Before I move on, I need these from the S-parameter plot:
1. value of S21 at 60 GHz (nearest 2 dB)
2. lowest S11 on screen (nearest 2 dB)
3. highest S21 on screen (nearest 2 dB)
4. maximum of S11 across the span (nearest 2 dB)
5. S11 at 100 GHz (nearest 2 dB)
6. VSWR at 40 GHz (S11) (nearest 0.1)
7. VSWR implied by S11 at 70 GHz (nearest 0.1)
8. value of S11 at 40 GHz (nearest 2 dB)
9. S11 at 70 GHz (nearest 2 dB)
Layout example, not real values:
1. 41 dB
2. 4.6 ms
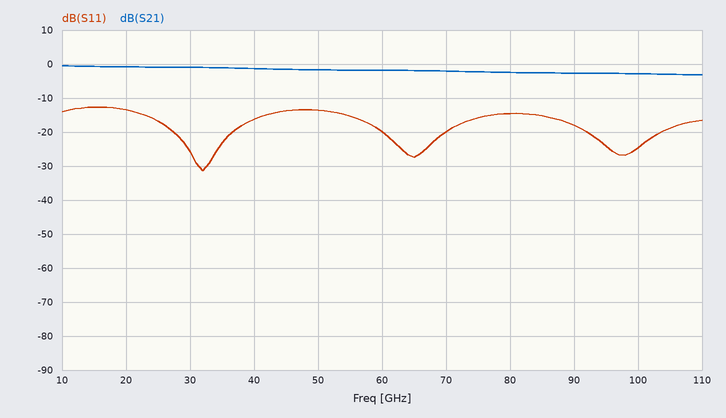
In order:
1. -2 dB
2. -32 dB
3. 0 dB
4. -12 dB
5. -24 dB
6. 1.4
7. 1.2
8. -16 dB
9. -20 dB
